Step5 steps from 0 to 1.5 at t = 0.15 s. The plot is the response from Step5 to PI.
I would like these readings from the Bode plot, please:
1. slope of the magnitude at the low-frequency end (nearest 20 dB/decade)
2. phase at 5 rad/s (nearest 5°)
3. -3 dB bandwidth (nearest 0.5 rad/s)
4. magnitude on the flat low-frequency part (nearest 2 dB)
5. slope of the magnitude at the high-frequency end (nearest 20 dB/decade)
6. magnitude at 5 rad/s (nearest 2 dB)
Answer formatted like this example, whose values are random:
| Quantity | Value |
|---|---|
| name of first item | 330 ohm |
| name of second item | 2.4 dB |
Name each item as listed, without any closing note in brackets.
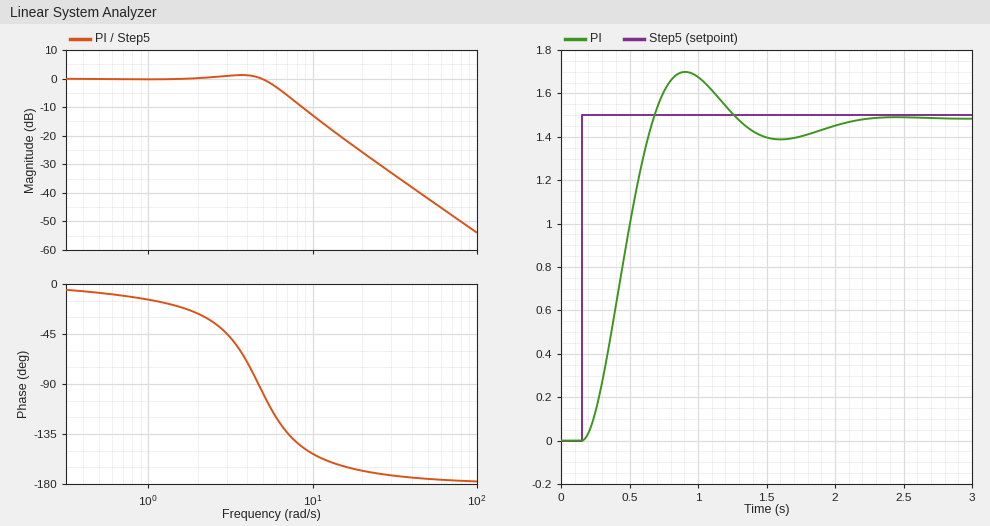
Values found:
| Quantity | Value |
|---|---|
| slope of the magnitude at the low-frequency end | 0 dB/decade |
| phase at 5 rad/s | -100° |
| -3 dB bandwidth | 6.0 rad/s |
| magnitude on the flat low-frequency part | 0 dB |
| slope of the magnitude at the high-frequency end | -40 dB/decade |
| magnitude at 5 rad/s | 0 dB |
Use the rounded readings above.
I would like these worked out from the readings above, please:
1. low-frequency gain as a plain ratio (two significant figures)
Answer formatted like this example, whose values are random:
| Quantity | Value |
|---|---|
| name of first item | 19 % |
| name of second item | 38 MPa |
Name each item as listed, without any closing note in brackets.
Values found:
| Quantity | Value |
|---|---|
| low-frequency gain as a plain ratio | 1.0 |
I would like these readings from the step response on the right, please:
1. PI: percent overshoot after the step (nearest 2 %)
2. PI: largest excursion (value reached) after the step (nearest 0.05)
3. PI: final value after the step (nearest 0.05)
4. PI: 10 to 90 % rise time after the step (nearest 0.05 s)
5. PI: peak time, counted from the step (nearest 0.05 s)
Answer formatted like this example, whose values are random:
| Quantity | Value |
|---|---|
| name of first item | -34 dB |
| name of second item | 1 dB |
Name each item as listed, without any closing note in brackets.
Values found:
| Quantity | Value |
|---|---|
| PI: percent overshoot after the step | 14 % |
| PI: largest excursion (value reached) after the step | 1.70 |
| PI: final value after the step | 1.50 |
| PI: 10 to 90 % rise time after the step | 0.35 s |
| PI: peak time, counted from the step | 0.75 s |
